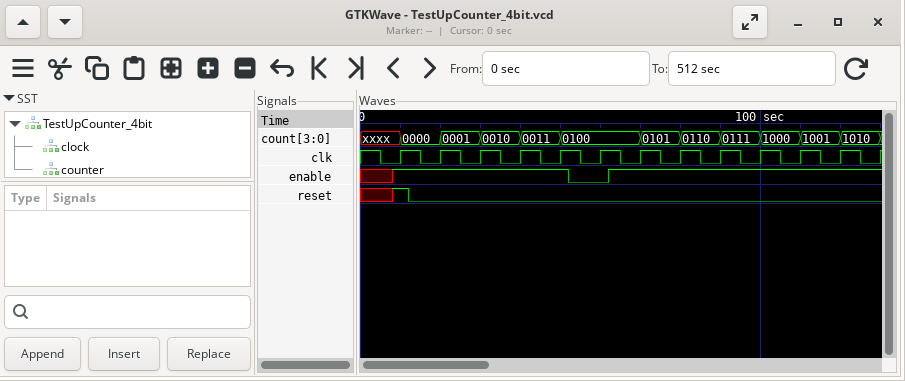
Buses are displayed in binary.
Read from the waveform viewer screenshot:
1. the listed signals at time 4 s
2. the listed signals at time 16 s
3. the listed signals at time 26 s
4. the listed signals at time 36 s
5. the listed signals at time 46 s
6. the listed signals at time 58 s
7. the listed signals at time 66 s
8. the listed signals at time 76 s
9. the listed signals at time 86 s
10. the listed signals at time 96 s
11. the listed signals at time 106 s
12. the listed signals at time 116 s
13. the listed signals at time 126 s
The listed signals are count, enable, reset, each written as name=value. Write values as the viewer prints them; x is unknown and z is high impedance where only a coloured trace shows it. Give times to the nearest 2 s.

count=xxxx, enable=x, reset=x
count=0000, enable=1, reset=0
count=0001, enable=1, reset=0
count=0010, enable=1, reset=0
count=0011, enable=1, reset=0
count=0100, enable=0, reset=0
count=0100, enable=1, reset=0
count=0101, enable=1, reset=0
count=0110, enable=1, reset=0
count=0111, enable=1, reset=0
count=1000, enable=1, reset=0
count=1001, enable=1, reset=0
count=1010, enable=1, reset=0
